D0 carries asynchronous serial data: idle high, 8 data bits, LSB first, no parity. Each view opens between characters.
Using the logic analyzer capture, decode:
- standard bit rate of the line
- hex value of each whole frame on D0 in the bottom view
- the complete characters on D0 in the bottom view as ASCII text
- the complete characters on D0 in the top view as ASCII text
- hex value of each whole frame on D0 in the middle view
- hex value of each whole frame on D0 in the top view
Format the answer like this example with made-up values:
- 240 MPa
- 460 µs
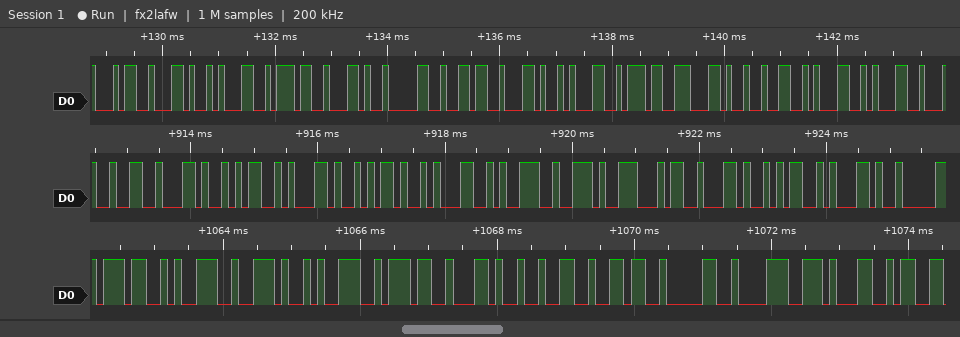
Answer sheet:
- 9600 baud
- 37, 39, 2E, 39, 37, 2C, 32, 36, 30, 38, 31
- "79.97,26081"
- "4,17,06,17,211"
- 32, 2C, 4D, 2C, 2D, 31, 39, 2E, 34, 2C, 4D, 2C
- 34, 2C, 31, 37, 2C, 30, 36, 2C, 31, 37, 2C, 32, 31, 31
